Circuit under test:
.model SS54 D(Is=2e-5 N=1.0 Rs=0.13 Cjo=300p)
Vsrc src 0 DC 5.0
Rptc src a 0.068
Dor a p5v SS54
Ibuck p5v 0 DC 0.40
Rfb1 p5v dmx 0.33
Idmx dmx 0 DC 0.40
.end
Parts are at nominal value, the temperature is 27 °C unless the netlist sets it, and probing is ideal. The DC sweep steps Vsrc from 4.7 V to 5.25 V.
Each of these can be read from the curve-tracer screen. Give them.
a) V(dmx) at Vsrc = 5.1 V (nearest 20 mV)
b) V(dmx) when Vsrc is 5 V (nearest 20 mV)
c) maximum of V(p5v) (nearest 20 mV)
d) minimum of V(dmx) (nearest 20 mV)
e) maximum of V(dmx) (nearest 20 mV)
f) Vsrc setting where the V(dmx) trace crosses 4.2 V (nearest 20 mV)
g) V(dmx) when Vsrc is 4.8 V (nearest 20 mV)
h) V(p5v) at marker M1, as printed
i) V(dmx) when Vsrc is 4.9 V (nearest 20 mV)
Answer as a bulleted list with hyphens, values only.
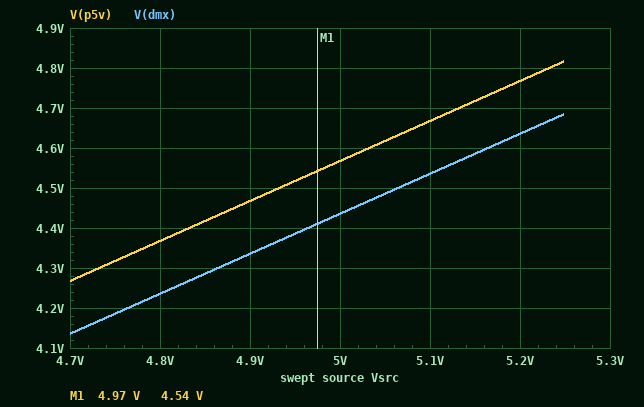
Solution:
- 4.54 V
- 4.44 V
- 4.82 V
- 4.14 V
- 4.68 V
- 4.76 V
- 4.24 V
- 4.54 V
- 4.34 V
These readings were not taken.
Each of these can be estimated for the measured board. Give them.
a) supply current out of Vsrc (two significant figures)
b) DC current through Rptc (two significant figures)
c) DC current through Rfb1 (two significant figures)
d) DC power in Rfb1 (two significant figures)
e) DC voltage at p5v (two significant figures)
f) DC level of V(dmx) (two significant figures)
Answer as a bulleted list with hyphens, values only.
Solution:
- 800 mA
- 800 mA
- 400 mA
- 53 mW
- 4.6 V
- 4.4 V
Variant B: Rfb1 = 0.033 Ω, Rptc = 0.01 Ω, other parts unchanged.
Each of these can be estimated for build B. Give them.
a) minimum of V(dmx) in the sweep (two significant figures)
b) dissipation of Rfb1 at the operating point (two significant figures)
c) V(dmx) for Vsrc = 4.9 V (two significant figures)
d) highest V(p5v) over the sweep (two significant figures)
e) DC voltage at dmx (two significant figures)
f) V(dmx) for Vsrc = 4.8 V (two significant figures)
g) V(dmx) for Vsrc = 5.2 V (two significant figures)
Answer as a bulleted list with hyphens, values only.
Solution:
- 4.3 V
- 5.3 mW
- 4.5 V
- 4.9 V
- 4.6 V
- 4.4 V
- 4.8 V
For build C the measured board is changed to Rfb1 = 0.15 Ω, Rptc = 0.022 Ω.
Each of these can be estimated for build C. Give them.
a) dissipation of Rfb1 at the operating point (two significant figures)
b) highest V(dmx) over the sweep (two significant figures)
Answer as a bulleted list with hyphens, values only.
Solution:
- 24 mW
- 4.8 V
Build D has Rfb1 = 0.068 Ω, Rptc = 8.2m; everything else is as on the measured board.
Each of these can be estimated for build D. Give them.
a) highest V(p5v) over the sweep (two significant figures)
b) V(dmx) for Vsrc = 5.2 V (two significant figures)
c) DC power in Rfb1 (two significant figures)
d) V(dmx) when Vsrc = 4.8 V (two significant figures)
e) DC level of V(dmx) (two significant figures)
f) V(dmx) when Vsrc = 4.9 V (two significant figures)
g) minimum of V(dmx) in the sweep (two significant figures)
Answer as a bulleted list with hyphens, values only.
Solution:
- 4.9 V
- 4.8 V
- 11 mW
- 4.4 V
- 4.6 V
- 4.5 V
- 4.3 V
